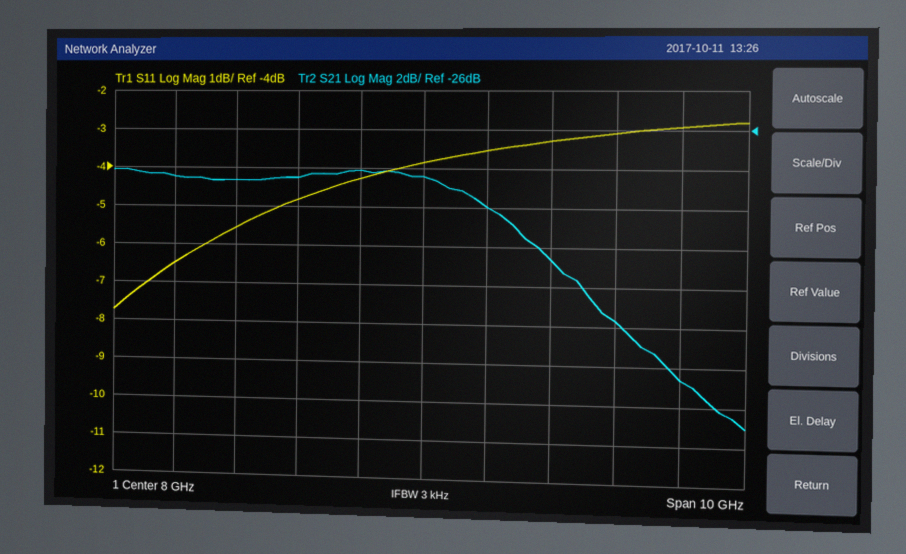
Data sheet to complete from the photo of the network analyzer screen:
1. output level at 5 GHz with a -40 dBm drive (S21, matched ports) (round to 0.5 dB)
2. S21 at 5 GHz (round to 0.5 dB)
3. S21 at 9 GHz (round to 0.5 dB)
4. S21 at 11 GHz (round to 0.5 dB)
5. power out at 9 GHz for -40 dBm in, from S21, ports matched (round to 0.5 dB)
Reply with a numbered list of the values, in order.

1. -68.5 dBm
2. -28.5 dB
3. -30.0 dB
4. -35.5 dB
5. -70.0 dBm
